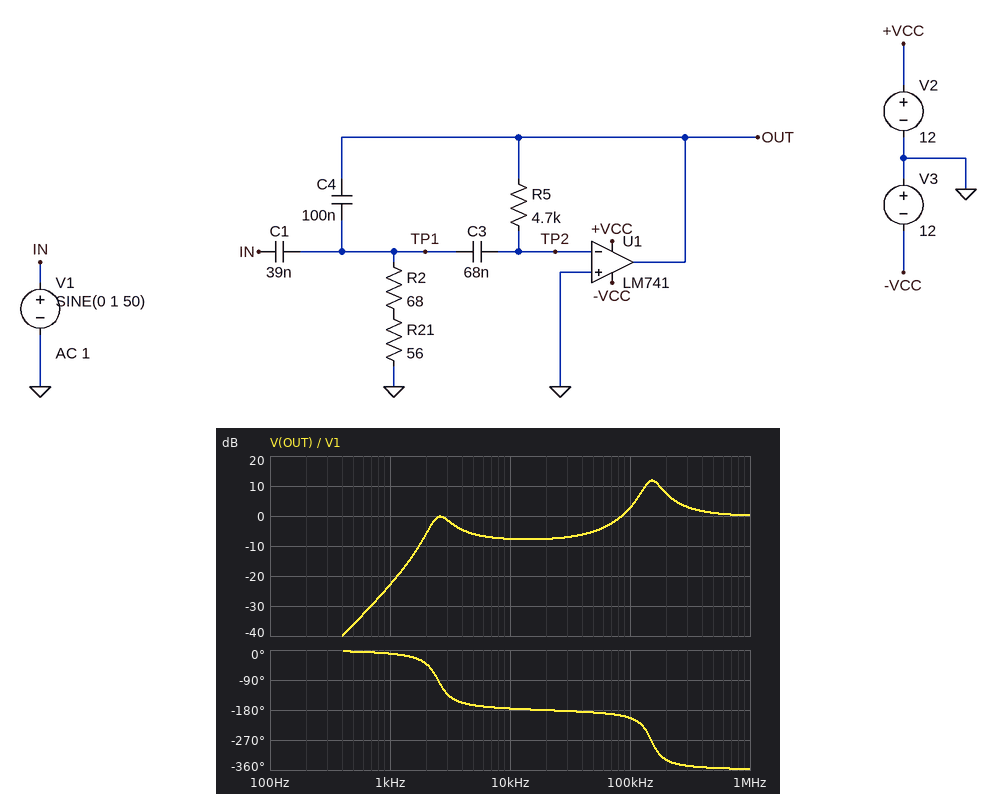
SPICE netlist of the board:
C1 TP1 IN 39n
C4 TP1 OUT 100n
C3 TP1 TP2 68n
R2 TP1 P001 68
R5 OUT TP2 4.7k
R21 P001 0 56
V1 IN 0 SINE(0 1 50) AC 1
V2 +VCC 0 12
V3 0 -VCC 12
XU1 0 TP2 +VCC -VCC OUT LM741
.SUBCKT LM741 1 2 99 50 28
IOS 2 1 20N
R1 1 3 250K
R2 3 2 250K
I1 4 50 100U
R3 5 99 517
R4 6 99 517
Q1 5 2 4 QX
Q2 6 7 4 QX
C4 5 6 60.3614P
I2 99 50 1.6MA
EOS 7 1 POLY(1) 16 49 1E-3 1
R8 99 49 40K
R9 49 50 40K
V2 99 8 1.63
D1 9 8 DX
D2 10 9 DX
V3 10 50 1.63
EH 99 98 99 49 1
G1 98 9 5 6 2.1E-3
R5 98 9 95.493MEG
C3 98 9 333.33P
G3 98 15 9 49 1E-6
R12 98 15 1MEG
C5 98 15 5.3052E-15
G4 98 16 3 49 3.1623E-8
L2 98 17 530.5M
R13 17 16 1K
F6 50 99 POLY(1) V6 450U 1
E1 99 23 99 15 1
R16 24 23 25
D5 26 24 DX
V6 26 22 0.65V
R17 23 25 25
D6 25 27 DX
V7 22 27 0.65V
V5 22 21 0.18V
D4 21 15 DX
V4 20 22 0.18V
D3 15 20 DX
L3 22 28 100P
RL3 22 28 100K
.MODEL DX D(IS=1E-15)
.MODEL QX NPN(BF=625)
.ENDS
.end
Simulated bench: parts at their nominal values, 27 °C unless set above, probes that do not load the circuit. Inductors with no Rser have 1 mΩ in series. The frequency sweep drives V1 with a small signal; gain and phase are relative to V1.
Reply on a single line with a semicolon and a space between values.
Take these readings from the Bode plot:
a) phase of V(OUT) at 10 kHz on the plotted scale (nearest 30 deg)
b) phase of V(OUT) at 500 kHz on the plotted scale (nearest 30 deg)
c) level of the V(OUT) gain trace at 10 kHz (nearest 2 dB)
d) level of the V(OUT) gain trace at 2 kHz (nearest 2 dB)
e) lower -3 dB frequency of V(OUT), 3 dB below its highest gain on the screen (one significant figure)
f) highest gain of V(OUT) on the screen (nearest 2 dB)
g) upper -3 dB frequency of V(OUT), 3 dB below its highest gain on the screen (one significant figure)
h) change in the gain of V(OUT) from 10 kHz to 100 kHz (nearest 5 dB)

-180 deg; -360 deg; -8 dB; -6 dB; 100 kHz; 12 dB; 200 kHz; 10 dB
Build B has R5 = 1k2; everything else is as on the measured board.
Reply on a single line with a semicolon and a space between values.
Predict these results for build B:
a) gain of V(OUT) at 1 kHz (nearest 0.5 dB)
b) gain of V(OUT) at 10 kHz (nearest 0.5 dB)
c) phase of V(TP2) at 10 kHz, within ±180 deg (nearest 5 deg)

-36.0 dB; -6.5 dB; 155 deg
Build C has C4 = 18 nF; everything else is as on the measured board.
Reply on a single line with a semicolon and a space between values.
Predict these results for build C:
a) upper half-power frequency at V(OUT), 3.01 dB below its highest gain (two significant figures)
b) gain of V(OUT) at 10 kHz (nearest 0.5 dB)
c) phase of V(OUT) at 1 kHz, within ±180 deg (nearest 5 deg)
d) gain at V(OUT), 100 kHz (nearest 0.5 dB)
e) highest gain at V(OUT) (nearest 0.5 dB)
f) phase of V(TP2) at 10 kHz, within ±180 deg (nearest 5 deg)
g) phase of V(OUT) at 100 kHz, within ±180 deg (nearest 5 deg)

200 kHz; 9.0 dB; -5 deg; 11.0 dB; 14.0 dB; 125 deg; 145 deg
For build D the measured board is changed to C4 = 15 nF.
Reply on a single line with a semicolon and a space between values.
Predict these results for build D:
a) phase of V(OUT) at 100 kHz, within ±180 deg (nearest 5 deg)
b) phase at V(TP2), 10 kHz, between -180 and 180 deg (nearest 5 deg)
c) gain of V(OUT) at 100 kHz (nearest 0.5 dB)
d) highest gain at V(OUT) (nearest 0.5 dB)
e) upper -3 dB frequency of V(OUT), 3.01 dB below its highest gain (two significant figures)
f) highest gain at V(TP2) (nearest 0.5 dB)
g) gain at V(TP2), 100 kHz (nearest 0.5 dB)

145 deg; 130 deg; 12.0 dB; 14.5 dB; 200 kHz; 4.5 dB; -3.5 dB
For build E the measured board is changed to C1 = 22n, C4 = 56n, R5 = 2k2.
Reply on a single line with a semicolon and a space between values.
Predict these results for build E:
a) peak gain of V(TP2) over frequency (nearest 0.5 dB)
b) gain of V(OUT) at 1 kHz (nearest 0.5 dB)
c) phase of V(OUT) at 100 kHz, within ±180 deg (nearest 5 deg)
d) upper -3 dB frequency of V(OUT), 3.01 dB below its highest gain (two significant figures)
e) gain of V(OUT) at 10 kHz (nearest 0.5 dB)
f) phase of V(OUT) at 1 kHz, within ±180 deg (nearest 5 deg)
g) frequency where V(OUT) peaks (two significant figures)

7.0 dB; -35.5 dB; 160 deg; 270 kHz; -6.5 dB; -5 deg; 210 kHz
